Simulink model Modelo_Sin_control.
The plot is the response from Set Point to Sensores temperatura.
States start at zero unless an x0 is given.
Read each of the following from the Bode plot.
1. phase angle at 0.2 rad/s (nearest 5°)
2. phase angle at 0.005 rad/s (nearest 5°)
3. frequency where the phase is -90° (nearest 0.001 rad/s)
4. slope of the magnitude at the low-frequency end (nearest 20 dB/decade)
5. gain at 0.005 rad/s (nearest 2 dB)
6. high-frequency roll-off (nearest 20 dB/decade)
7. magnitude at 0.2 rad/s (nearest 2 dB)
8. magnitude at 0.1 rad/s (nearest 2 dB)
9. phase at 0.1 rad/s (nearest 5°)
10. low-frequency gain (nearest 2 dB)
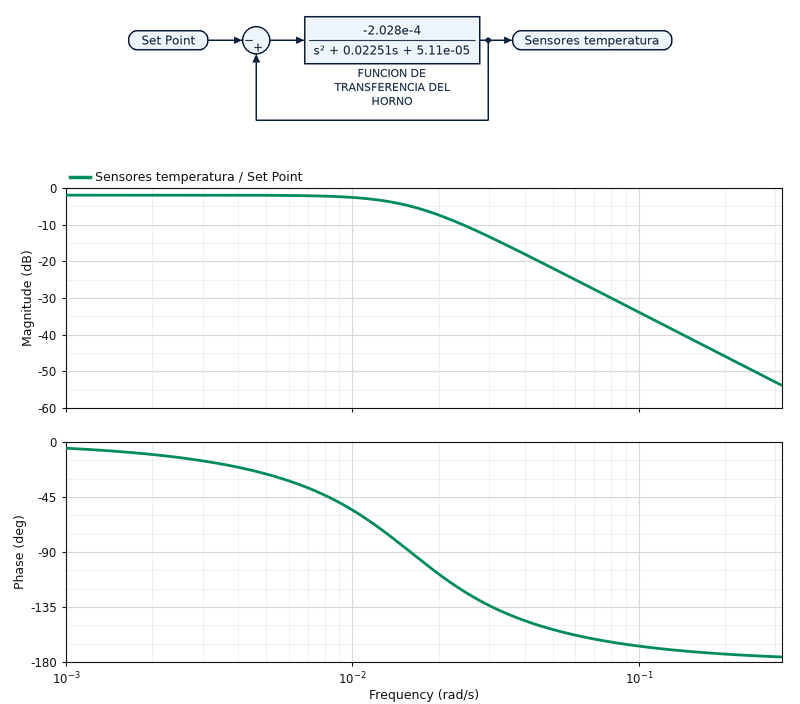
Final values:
-175°
-25°
0.016 rad/s
0 dB/decade
-2 dB
-40 dB/decade
-46 dB
-34 dB
-165°
-2 dB
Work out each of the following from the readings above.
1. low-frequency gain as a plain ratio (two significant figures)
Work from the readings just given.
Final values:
0.79
